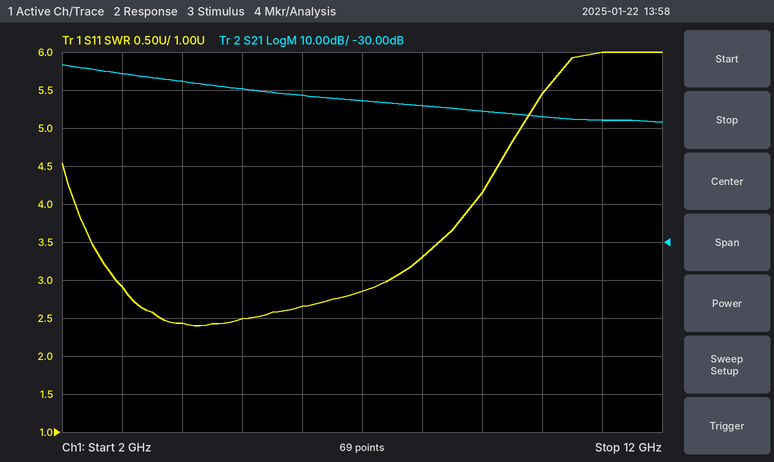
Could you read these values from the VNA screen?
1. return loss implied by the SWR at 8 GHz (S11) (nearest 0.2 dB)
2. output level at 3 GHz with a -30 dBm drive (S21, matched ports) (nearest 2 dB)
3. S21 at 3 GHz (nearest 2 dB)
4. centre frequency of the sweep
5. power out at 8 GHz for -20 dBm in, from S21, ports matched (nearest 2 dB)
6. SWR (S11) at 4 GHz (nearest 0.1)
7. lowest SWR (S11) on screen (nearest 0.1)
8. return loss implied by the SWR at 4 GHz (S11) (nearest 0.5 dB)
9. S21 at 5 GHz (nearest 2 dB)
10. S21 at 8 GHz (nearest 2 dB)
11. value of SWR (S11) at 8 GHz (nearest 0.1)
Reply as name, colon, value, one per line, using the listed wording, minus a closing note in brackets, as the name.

return loss implied by the SWR at 8 GHz (S11): 5.4 dB
output level at 3 GHz with a -30 dBm drive (S21, matched ports): -16 dBm
S21 at 3 GHz: 14 dB
centre frequency of the sweep: 7 GHz
power out at 8 GHz for -20 dBm in, from S21, ports matched: -14 dBm
SWR (S11) at 4 GHz: 2.4
lowest SWR (S11) on screen: 2.4
return loss implied by the SWR at 4 GHz (S11): 7.5 dB
S21 at 5 GHz: 10 dB
S21 at 8 GHz: 6 dB
value of SWR (S11) at 8 GHz: 3.3
